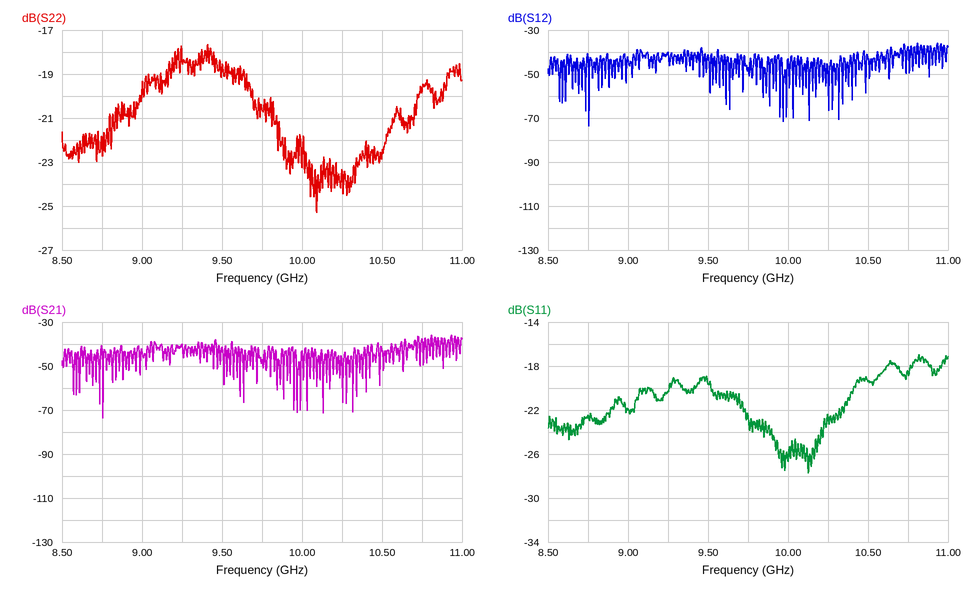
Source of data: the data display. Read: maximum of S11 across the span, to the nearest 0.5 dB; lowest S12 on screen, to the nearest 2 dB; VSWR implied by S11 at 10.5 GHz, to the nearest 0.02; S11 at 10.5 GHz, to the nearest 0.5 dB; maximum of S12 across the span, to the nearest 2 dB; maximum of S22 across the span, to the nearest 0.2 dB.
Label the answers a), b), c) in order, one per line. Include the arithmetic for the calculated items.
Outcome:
a) -17.0 dB
b) -74 dB
c) |Γ| = 10^(-19.5/20) = 0.1059; VSWR = (1 + 0.1059)/(1 − 0.1059) ≈ 1.24
d) -19.5 dB
e) -36 dB
f) -17.6 dB
